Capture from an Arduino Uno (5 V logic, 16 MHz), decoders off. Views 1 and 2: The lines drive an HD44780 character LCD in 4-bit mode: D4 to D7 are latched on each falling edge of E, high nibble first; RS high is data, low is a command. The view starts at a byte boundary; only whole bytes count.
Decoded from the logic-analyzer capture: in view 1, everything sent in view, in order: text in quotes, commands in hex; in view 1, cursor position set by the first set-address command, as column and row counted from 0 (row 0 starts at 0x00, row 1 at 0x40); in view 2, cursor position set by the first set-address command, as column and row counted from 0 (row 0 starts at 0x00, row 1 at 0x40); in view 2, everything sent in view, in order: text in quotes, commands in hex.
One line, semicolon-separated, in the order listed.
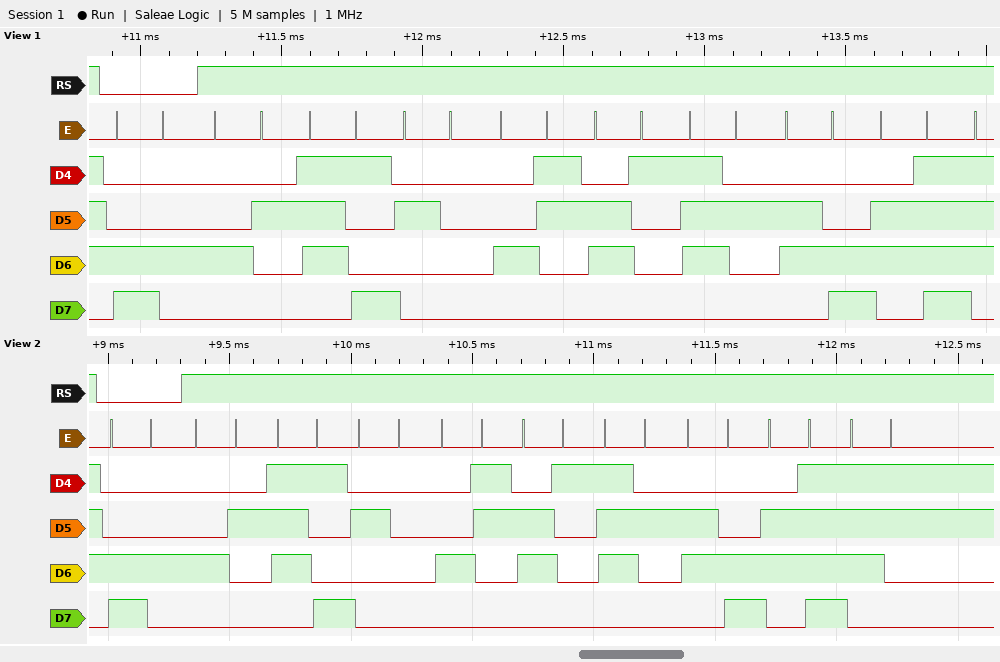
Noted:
0xC4 "By Carlo"; column 4, row 1; column 4, row 1; 0xC4 "By Carlos"
